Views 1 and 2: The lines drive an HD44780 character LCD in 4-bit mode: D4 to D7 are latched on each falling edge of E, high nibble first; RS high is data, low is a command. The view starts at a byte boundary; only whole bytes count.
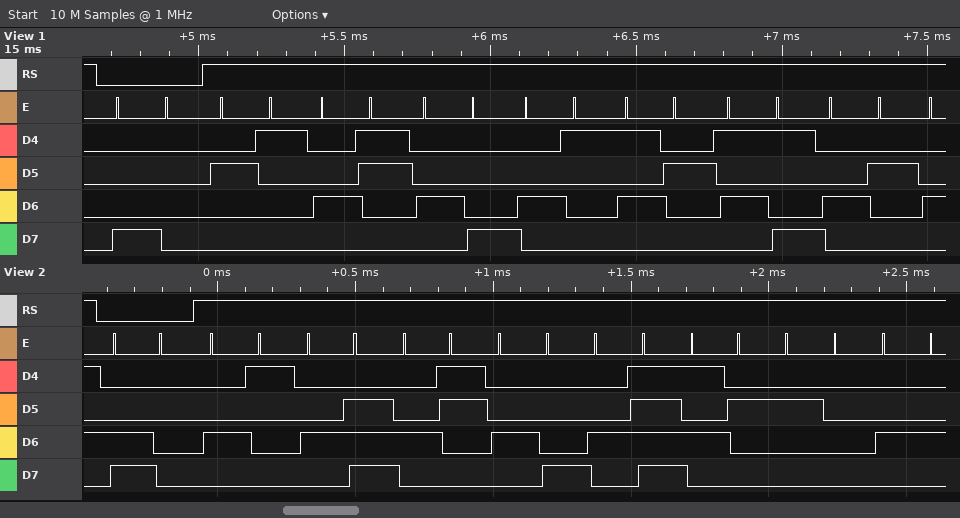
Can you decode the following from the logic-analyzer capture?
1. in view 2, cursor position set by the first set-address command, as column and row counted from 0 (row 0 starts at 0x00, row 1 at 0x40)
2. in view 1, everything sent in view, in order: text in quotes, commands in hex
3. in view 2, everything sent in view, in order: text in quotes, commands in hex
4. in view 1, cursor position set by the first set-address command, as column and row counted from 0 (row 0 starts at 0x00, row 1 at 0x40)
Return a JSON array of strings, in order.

["column 0, row 1", "0x80 \"!CHARYB\"", "0xC0 \"ANCHOR D\"", "column 0, row 0"]
